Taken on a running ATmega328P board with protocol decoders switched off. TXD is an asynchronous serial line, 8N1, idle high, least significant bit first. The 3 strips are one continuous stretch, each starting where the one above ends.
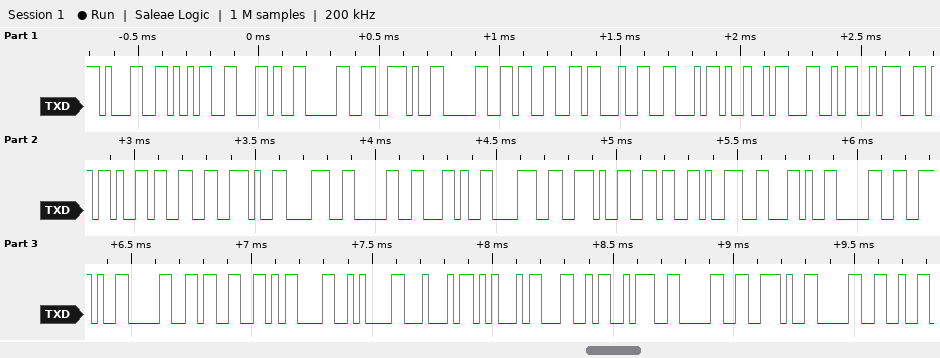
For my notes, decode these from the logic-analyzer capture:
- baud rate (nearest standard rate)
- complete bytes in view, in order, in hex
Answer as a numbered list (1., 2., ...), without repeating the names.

1. 38400 baud
2. 31 35 2C 30 2E 30 33 23 46 49 4C 3A 2D 33 2E 38 30 2C 38 2E 36 39 2C 30 2E 30 33 0D 0A 44 45 4C 3A 30 2E 30
